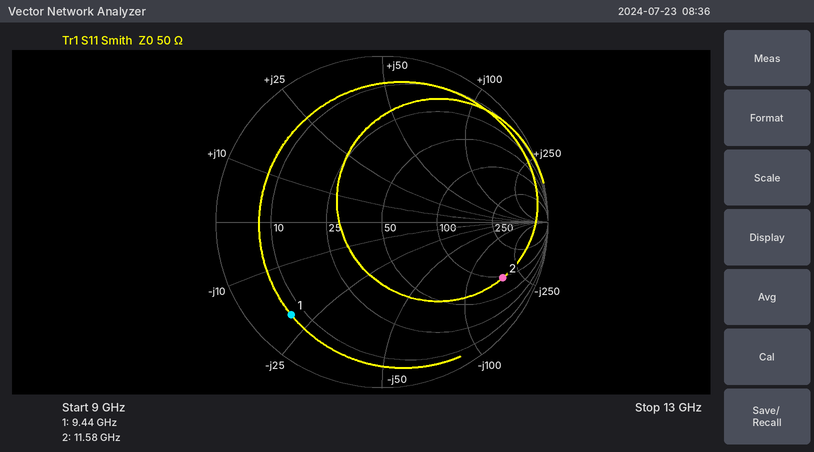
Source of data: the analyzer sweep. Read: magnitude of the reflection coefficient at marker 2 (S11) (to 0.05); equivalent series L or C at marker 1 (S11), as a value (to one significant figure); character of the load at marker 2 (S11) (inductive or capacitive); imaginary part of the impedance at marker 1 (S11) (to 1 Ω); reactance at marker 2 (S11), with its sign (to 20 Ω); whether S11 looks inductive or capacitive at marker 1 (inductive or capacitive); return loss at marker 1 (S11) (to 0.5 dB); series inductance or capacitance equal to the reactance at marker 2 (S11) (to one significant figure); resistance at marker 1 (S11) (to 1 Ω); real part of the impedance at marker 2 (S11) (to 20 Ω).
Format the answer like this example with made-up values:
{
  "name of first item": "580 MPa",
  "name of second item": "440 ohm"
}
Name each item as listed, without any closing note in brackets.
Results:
{
  "magnitude of the reflection coefficient at marker 2 (S11)": "0.80",
  "equivalent series L or C at marker 1 (S11), as a value": "800 fF",
  "character of the load at marker 2 (S11)": "capacitive",
  "imaginary part of the impedance at marker 1 (S11)": "-21 Ω",
  "reactance at marker 2 (S11), with its sign": "-180 Ω",
  "whether S11 looks inductive or capacitive at marker 1": "capacitive",
  "return loss at marker 1 (S11)": "2.0 dB",
  "series inductance or capacitance equal to the reactance at marker 2 (S11)": "80 fF",
  "resistance at marker 1 (S11)": "7 Ω",
  "real part of the impedance at marker 2 (S11)": "100 Ω"
}
